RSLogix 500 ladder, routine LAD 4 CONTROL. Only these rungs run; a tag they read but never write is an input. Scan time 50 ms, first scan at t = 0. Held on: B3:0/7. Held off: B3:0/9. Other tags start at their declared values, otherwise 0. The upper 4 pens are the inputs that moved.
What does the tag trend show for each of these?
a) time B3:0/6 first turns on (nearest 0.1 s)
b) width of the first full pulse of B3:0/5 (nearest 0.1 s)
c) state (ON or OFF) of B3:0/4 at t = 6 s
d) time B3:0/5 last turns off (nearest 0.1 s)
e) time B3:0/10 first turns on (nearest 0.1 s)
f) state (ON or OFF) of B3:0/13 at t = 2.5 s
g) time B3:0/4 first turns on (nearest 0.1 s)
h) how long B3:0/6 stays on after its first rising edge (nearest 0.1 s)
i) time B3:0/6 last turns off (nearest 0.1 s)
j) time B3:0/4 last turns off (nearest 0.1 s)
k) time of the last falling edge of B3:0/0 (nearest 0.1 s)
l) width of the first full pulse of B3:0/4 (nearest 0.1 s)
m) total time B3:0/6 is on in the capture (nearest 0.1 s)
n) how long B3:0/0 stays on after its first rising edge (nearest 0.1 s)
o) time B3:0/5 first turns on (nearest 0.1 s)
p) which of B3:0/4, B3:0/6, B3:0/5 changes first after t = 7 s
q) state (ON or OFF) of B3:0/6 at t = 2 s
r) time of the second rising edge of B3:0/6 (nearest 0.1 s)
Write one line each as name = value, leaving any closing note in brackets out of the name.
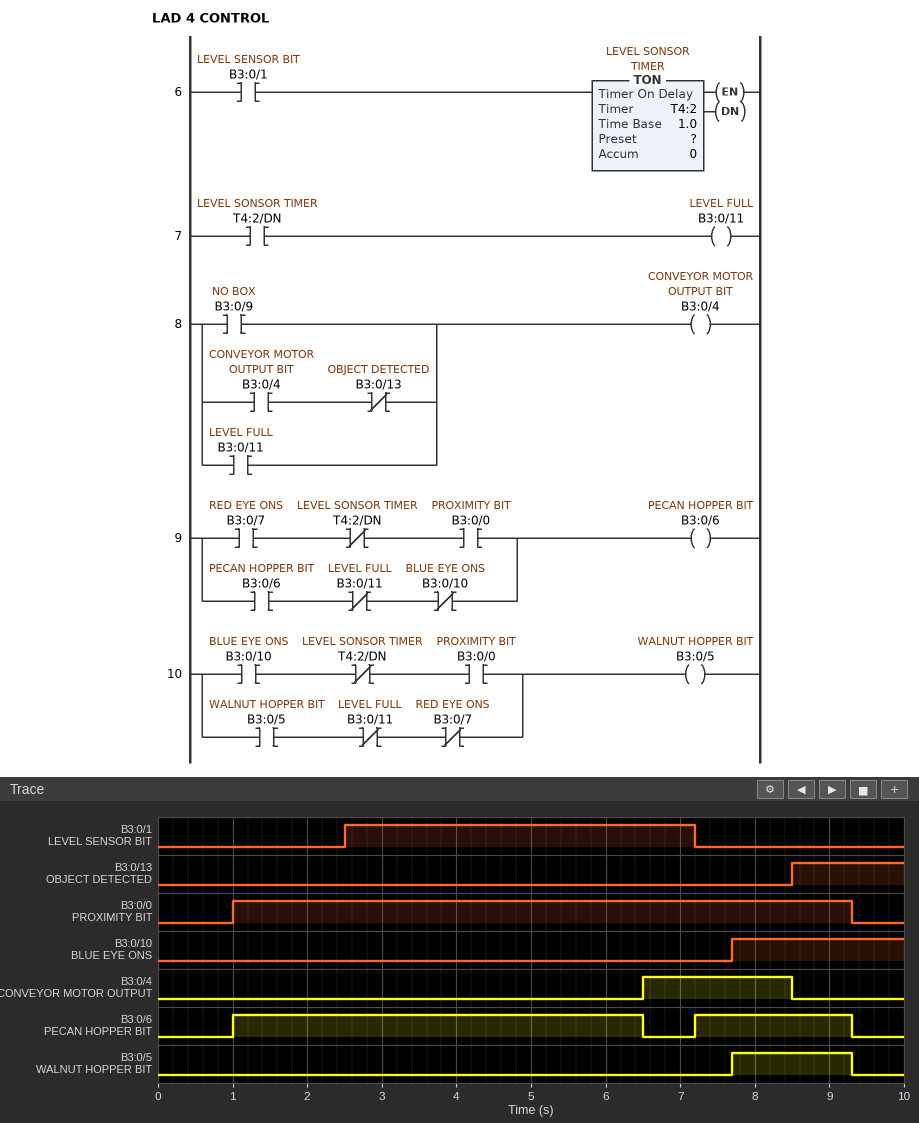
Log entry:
time B3:0/6 first turns on = 1.0 s
width of the first full pulse of B3:0/5 = 1.6 s
state (ON or OFF) of B3:0/4 at t = 6 s = OFF
time B3:0/5 last turns off = 9.3 s
time B3:0/10 first turns on = 7.7 s
state (ON or OFF) of B3:0/13 at t = 2.5 s = OFF
time B3:0/4 first turns on = 6.5 s
how long B3:0/6 stays on after its first rising edge = 5.5 s
time B3:0/6 last turns off = 9.3 s
time B3:0/4 last turns off = 8.5 s
time of the last falling edge of B3:0/0 = 9.3 s
width of the first full pulse of B3:0/4 = 2.0 s
total time B3:0/6 is on in the capture = 7.6 s
how long B3:0/0 stays on after its first rising edge = 8.3 s
time B3:0/5 first turns on = 7.7 s
which of B3:0/4, B3:0/6, B3:0/5 changes first after t = 7 s = B3:0/6
state (ON or OFF) of B3:0/6 at t = 2 s = ON
time of the second rising edge of B3:0/6 = 7.2 s
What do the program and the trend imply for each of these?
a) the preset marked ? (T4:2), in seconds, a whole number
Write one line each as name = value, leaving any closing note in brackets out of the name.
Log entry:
the preset marked ? (T4:2), in seconds, a whole number = 4 s
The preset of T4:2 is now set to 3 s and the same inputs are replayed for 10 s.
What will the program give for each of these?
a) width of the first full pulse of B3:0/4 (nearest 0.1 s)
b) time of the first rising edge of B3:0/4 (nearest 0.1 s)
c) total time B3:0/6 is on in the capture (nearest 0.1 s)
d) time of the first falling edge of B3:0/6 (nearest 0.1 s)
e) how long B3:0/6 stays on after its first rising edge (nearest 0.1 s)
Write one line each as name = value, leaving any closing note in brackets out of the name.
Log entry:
width of the first full pulse of B3:0/4 = 3.0 s
time of the first rising edge of B3:0/4 = 5.5 s
total time B3:0/6 is on in the capture = 6.6 s
time of the first falling edge of B3:0/6 = 5.5 s
how long B3:0/6 stays on after its first rising edge = 4.5 s
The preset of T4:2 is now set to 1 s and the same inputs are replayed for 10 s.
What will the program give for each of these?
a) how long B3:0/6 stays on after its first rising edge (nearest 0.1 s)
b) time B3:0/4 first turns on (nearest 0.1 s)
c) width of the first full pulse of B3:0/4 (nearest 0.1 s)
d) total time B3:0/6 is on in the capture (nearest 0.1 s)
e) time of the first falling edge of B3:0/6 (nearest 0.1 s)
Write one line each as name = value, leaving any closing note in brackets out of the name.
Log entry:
how long B3:0/6 stays on after its first rising edge = 2.5 s
time B3:0/4 first turns on = 3.5 s
width of the first full pulse of B3:0/4 = 5.0 s
total time B3:0/6 is on in the capture = 4.6 s
time of the first falling edge of B3:0/6 = 3.5 s
